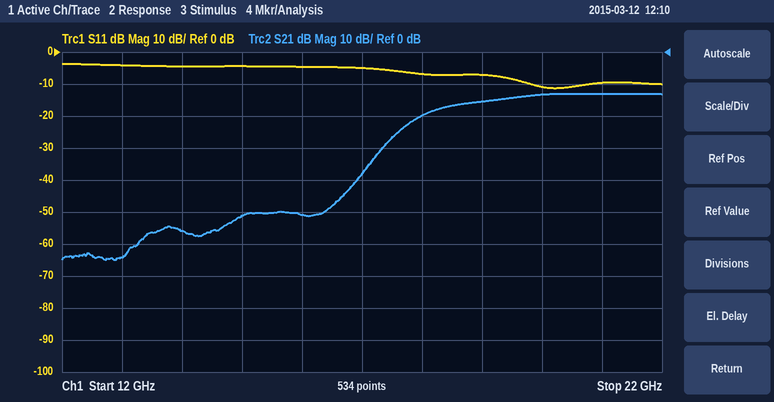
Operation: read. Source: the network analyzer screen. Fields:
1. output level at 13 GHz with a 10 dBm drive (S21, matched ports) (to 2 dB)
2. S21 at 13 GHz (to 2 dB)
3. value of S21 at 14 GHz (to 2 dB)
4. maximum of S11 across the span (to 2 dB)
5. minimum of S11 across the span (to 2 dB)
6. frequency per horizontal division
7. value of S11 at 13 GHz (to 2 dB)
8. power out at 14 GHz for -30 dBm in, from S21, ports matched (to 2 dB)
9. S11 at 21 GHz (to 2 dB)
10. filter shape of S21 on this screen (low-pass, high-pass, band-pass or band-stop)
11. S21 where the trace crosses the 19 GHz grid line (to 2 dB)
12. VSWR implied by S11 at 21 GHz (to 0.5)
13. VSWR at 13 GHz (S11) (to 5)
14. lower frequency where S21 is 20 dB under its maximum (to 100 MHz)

-54 dBm
-64 dB
-56 dB
-4 dB
-12 dB
1 GHz
-4 dB
-86 dBm
-10 dB
high-pass
-16 dB
2.0
5
17.2 GHz
